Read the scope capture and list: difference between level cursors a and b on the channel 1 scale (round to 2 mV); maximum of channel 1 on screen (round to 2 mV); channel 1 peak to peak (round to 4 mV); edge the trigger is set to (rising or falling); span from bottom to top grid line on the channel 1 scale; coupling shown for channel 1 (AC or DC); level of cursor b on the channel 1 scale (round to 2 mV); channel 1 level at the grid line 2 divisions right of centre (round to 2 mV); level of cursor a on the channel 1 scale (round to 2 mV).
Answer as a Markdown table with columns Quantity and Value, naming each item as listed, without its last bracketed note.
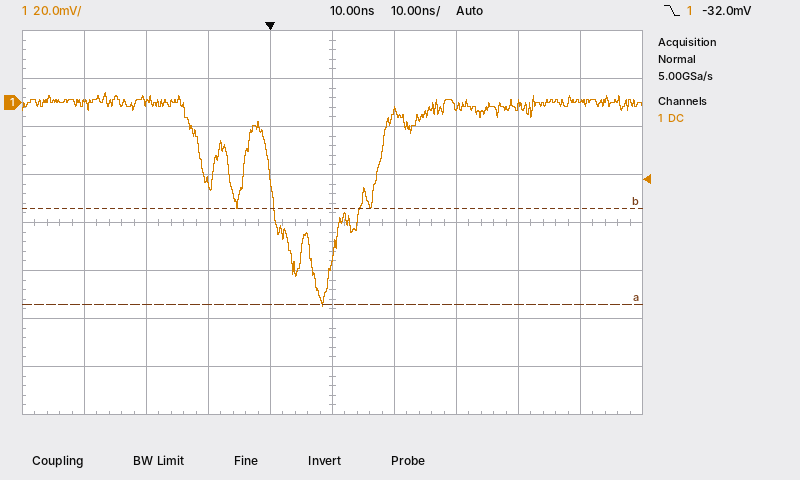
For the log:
| Quantity | Value |
|---|---|
| difference between level cursors a and b on the channel 1 scale | 40 mV |
| maximum of channel 1 on screen | 4 mV |
| channel 1 peak to peak | 88 mV |
| edge the trigger is set to | falling |
| span from bottom to top grid line on the channel 1 scale | 160 mV |
| coupling shown for channel 1 | DC |
| level of cursor b on the channel 1 scale | -44 mV |
| channel 1 level at the grid line 2 divisions right of centre | -2 mV |
| level of cursor a on the channel 1 scale | -84 mV |
